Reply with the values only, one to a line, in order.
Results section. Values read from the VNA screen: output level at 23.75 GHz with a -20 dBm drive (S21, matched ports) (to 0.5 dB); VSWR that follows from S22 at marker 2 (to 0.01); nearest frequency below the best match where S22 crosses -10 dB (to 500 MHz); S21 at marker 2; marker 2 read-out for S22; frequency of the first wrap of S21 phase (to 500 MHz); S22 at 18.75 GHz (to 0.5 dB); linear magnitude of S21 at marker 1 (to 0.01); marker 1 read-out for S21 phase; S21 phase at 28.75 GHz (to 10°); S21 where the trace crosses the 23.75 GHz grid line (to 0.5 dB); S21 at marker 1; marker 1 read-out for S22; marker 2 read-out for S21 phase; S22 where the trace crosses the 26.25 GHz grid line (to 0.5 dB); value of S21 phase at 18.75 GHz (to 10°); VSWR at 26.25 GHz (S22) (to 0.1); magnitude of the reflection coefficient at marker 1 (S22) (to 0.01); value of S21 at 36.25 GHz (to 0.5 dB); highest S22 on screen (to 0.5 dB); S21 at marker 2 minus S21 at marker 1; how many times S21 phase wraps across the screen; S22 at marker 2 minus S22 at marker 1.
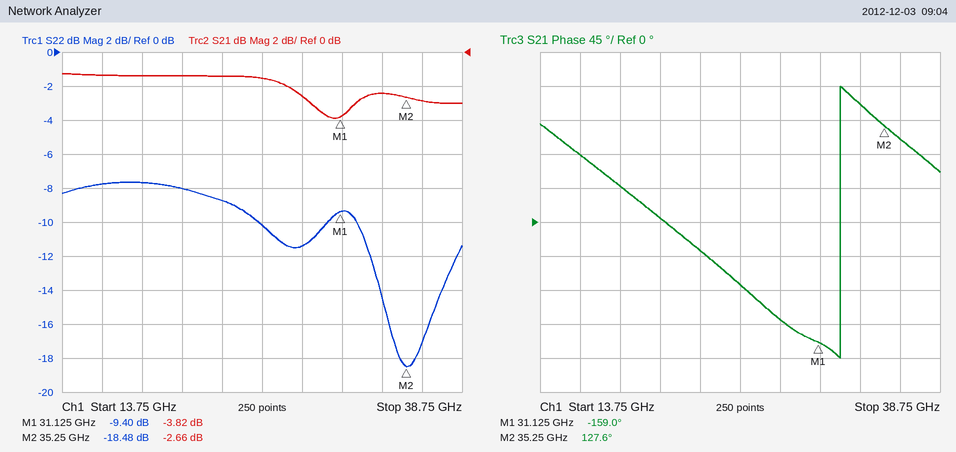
-21.5 dBm
1.27
32.0 GHz
-2.66 dB
-18.48 dB
32.5 GHz
-7.5 dB
0.64
-159.0°
-130°
-1.5 dB
-3.82 dB
-9.40 dB
127.6°
-10.0 dB
50°
1.9
0.34
-3.0 dB
-7.5 dB
1.16 dB
1
-9.08 dB
